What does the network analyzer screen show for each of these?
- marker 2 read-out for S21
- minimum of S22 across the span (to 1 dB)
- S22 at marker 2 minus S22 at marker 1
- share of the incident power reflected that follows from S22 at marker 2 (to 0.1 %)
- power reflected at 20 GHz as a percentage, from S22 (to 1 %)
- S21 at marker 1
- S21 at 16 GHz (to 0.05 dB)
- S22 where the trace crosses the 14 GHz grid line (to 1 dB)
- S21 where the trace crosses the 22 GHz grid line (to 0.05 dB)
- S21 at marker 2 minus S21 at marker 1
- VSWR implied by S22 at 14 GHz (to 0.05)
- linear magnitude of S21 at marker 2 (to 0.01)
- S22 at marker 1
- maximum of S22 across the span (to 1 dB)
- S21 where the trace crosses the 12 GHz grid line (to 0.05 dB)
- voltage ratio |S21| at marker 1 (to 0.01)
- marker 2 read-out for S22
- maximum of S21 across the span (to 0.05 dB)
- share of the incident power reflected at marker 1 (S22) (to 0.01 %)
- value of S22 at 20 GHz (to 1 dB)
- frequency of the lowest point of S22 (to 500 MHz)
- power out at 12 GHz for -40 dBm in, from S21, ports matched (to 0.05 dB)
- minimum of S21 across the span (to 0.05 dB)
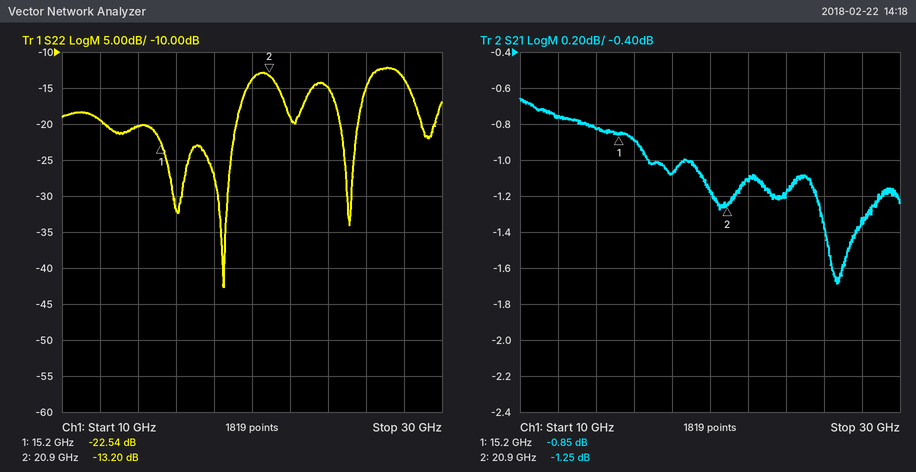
-1.25 dB
-43 dB
9.34 dB
4.8 %
4 %
-0.85 dB
-0.90 dB
-20 dB
-1.10 dB
-0.40 dB
1.20
0.87
-22.54 dB
-12 dB
-0.75 dB
0.91
-13.20 dB
-0.65 dB
0.56 %
-14 dB
18.5 GHz
-40.75 dBm
-1.70 dB
